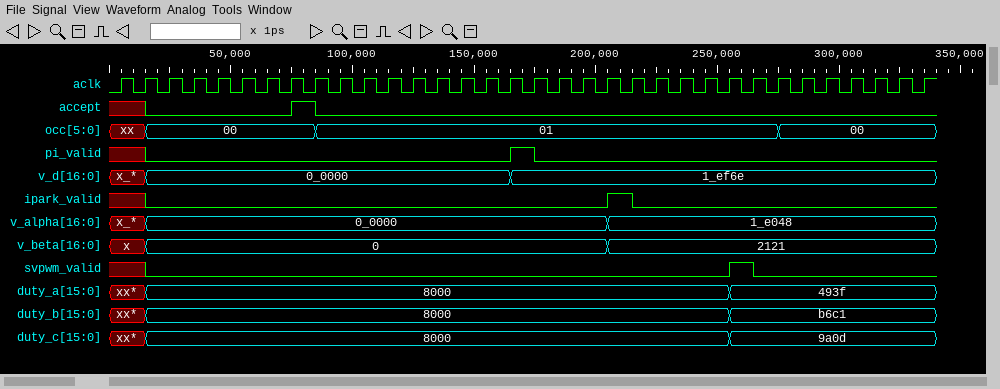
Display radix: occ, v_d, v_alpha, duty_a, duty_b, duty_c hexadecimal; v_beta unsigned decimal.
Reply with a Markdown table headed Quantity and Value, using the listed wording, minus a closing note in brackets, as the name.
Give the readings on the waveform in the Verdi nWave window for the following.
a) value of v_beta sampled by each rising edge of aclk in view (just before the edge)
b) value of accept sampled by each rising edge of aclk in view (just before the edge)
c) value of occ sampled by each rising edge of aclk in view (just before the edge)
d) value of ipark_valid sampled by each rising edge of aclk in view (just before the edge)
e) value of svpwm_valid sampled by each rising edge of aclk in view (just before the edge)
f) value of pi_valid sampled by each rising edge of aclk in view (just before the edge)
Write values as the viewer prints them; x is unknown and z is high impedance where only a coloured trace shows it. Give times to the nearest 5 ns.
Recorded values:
| Quantity | Value |
|---|---|
| value of v_beta sampled by each rising edge of aclk in view | x, x, 0, 0, 0, 0, 0, 0, 0, 0, 0, 0, 0, 0, 0, 0, 0, 0, 0, 0, 0, 2121, 2121, 2121, 2121, 2121, 2121, 2121, 2121, 2121, 2121, 2121, 2121, 2121 |
| value of accept sampled by each rising edge of aclk in view | x x 0 0 0 0 0 0 1 0 0 0 0 0 0 0 0 0 0 0 0 0 0 0 0 0 0 0 0 0 0 0 0 0 |
| value of occ sampled by each rising edge of aclk in view | xx, xx, 00, 00, 00, 00, 00, 00, 00, 01, 01, 01, 01, 01, 01, 01, 01, 01, 01, 01, 01, 01, 01, 01, 01, 01, 01, 01, 00, 00, 00, 00, 00, 00 |
| value of ipark_valid sampled by each rising edge of aclk in view | x x 0 0 0 0 0 0 0 0 0 0 0 0 0 0 0 0 0 0 0 1 0 0 0 0 0 0 0 0 0 0 0 0 |
| value of svpwm_valid sampled by each rising edge of aclk in view | x x 0 0 0 0 0 0 0 0 0 0 0 0 0 0 0 0 0 0 0 0 0 0 0 0 1 0 0 0 0 0 0 0 |
| value of pi_valid sampled by each rising edge of aclk in view | x x 0 0 0 0 0 0 0 0 0 0 0 0 0 0 0 1 0 0 0 0 0 0 0 0 0 0 0 0 0 0 0 0 |
